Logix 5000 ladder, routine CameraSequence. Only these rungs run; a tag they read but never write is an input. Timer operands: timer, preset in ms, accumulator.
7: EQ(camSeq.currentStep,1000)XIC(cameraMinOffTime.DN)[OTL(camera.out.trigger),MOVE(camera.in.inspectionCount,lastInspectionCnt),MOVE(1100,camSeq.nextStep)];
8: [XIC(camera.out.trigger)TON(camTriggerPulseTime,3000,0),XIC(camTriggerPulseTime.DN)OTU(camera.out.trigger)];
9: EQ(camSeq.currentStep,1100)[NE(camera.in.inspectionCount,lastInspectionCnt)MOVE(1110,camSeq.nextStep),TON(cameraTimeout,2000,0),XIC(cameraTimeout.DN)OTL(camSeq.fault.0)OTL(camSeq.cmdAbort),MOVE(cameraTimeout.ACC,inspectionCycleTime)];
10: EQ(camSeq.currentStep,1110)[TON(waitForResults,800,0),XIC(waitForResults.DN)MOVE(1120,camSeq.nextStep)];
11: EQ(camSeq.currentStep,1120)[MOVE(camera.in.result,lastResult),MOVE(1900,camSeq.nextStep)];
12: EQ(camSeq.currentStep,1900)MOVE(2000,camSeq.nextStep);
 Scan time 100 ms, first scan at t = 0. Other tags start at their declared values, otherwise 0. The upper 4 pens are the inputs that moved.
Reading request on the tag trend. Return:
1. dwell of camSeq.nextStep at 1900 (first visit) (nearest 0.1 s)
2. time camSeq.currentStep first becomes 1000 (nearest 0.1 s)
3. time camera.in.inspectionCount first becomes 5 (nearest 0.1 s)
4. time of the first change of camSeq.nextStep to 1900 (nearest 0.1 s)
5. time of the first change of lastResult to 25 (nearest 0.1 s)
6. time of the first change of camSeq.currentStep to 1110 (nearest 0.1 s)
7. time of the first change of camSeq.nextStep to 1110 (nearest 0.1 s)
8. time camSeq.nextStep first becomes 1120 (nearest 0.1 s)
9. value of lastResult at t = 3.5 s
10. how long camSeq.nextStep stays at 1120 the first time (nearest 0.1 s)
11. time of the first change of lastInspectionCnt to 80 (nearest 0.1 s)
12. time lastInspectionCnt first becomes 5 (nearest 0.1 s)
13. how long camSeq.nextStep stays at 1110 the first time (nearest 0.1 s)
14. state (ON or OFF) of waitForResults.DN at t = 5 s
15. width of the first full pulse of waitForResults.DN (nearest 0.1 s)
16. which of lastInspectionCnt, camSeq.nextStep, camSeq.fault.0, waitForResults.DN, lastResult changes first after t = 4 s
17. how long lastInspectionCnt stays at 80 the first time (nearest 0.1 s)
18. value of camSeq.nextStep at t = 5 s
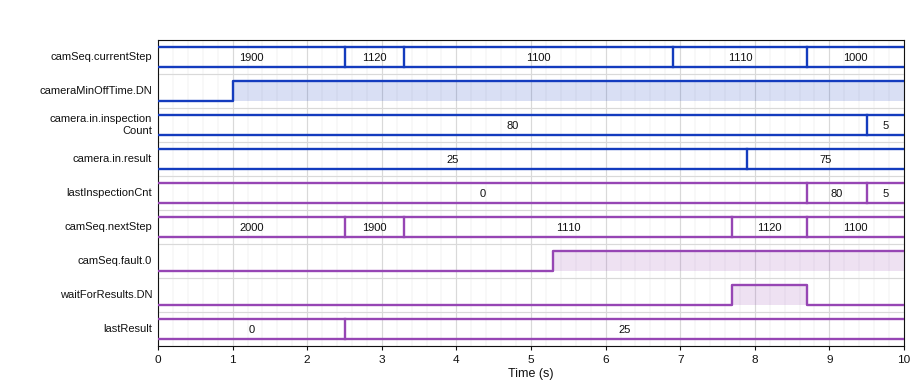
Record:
0.8 s
8.7 s
9.5 s
2.5 s
2.5 s
6.9 s
3.3 s
7.7 s
25
1.0 s
8.7 s
9.5 s
4.4 s
OFF
1.0 s
camSeq.fault.0
0.8 s
1110
